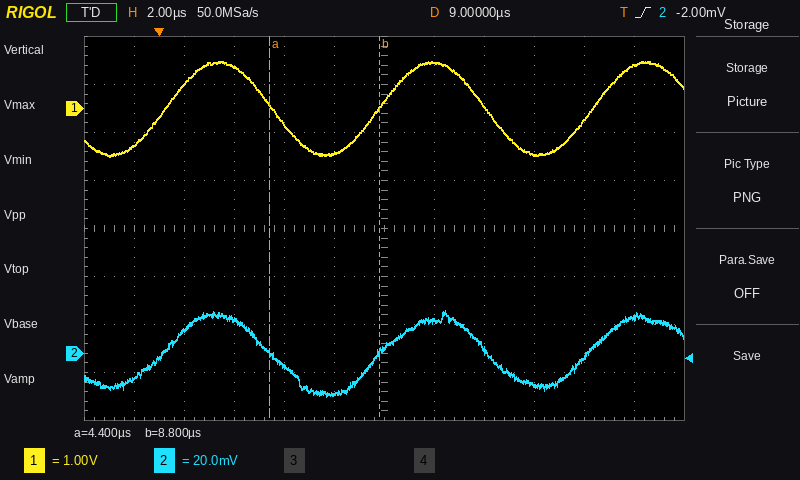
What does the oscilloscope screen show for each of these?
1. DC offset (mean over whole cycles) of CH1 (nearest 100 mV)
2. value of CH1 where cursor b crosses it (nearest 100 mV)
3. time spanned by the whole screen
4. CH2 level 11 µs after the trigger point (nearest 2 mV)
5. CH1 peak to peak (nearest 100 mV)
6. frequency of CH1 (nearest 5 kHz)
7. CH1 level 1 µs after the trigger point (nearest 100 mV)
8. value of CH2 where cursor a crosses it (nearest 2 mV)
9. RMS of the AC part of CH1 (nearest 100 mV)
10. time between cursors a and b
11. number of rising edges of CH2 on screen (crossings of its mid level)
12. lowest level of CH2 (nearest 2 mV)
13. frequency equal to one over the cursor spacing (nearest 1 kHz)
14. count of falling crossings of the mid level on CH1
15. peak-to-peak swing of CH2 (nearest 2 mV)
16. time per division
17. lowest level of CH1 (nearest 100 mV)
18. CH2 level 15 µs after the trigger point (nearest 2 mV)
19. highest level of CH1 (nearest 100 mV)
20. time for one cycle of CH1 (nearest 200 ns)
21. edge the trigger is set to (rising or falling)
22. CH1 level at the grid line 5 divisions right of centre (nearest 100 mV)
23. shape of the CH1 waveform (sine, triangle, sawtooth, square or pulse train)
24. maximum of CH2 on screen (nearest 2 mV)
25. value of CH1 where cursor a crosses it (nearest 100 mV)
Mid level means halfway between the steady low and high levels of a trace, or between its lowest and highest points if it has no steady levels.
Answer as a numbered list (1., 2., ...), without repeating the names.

1. 0.0 V
2. 0.0 V
3. 24 µs
4. 14 mV
5. 2.0 V
6. 115 kHz
7. 500 mV
8. 0 mV
9. 700 mV
10. 4.4 µs
11. 3
12. -18 mV
13. 227 kHz
14. 2
15. 36 mV
16. 2 µs
17. -1.0 V
18. -14 mV
19. 1.0 V
20. 8.6 µs
21. rising
22. 900 mV
23. sine
24. 18 mV
25. 100 mV
